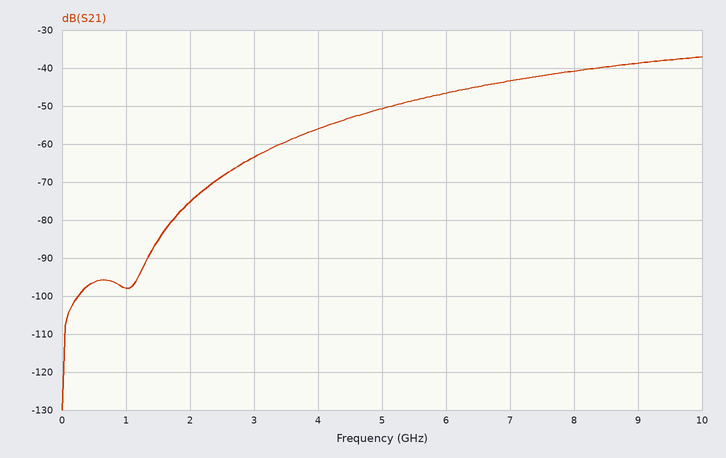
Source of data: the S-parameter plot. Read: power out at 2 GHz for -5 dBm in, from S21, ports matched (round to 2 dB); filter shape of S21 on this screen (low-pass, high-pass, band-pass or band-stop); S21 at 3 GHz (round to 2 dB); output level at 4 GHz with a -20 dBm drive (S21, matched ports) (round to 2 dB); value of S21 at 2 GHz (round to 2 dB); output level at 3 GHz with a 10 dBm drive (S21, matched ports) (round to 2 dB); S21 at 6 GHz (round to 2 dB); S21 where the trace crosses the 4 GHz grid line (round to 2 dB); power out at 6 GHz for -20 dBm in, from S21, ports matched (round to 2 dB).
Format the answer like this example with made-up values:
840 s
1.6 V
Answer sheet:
-80 dBm
high-pass
-64 dB
-76 dBm
-76 dB
-54 dBm
-46 dB
-56 dB
-66 dBm
